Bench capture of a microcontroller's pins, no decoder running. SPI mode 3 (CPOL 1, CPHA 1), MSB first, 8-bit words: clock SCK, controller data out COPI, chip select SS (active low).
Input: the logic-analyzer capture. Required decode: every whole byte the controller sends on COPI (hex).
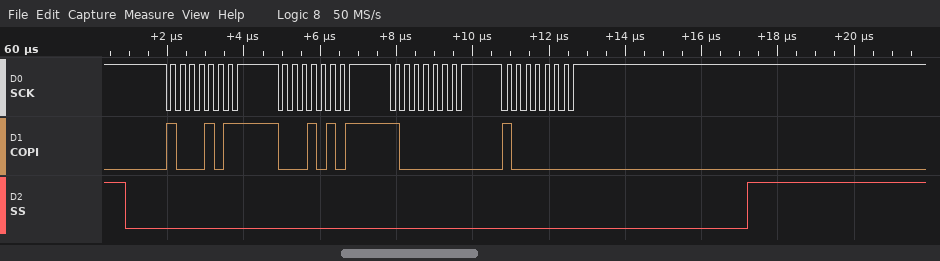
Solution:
8B 15 80 80
